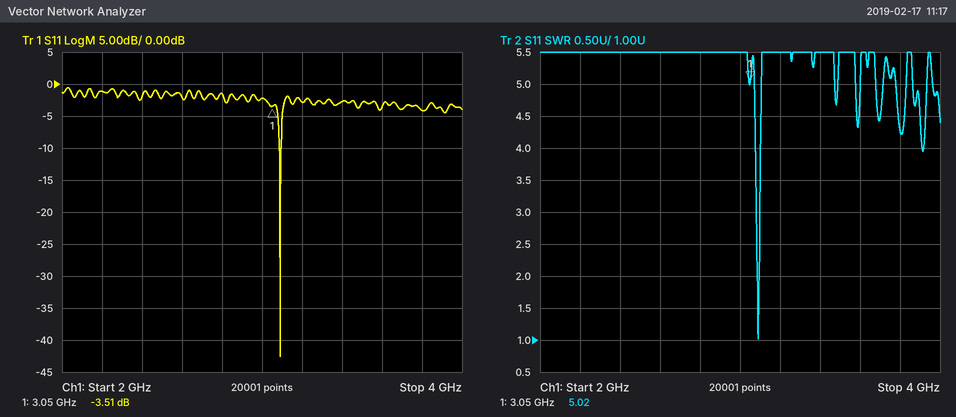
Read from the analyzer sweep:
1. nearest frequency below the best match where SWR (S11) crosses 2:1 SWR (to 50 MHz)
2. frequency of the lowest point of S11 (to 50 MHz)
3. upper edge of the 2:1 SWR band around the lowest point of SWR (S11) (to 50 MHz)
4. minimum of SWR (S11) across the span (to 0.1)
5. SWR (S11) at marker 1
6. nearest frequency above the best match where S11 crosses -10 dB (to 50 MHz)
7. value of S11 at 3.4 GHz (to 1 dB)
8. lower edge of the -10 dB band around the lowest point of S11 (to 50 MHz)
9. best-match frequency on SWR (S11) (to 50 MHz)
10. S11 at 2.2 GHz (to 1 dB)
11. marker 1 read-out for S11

3.10 GHz
3.10 GHz
3.10 GHz
1.0
5.02
3.10 GHz
-3 dB
3.10 GHz
3.10 GHz
-1 dB
-3.51 dB
